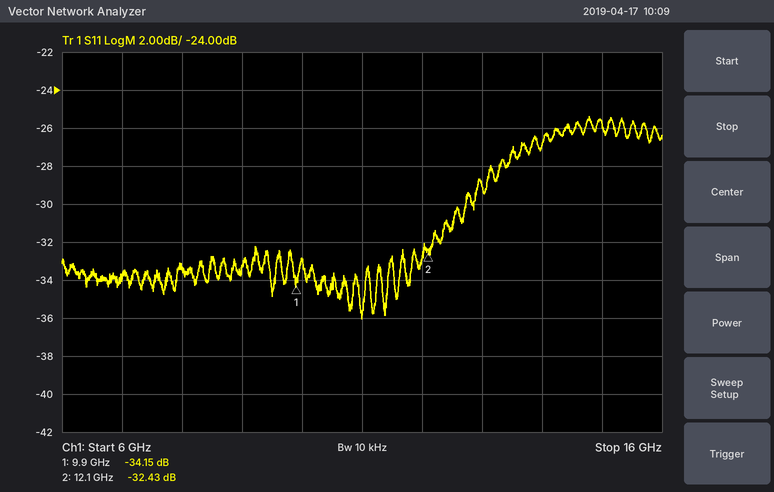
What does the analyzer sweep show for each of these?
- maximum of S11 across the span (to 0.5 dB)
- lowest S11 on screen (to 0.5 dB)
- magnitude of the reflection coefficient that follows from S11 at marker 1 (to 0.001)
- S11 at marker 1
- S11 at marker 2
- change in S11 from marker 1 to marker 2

-25.5 dB
-36.0 dB
0.020
-34.15 dB
-32.43 dB
1.72 dB
